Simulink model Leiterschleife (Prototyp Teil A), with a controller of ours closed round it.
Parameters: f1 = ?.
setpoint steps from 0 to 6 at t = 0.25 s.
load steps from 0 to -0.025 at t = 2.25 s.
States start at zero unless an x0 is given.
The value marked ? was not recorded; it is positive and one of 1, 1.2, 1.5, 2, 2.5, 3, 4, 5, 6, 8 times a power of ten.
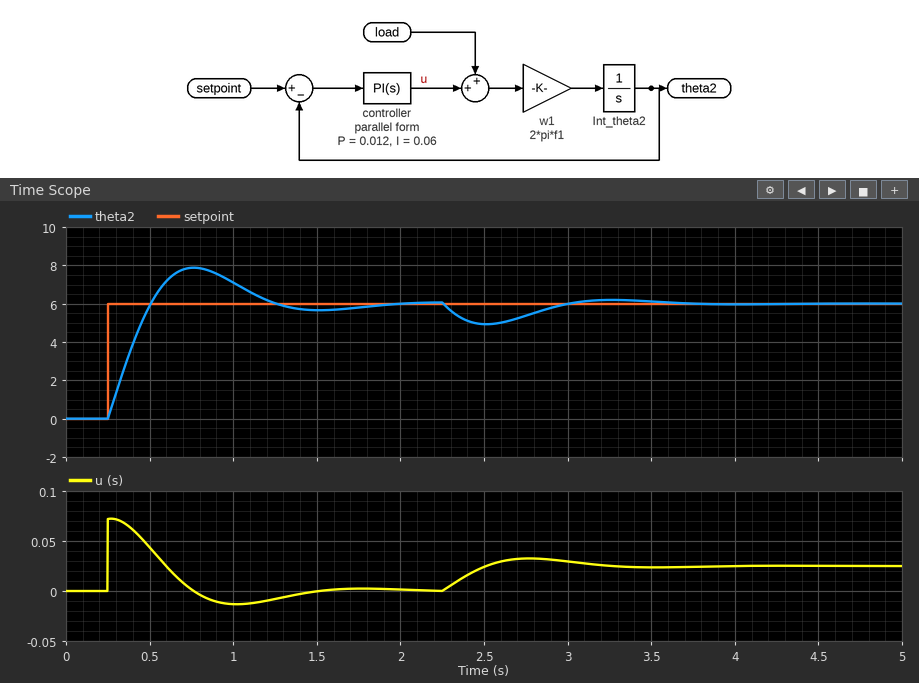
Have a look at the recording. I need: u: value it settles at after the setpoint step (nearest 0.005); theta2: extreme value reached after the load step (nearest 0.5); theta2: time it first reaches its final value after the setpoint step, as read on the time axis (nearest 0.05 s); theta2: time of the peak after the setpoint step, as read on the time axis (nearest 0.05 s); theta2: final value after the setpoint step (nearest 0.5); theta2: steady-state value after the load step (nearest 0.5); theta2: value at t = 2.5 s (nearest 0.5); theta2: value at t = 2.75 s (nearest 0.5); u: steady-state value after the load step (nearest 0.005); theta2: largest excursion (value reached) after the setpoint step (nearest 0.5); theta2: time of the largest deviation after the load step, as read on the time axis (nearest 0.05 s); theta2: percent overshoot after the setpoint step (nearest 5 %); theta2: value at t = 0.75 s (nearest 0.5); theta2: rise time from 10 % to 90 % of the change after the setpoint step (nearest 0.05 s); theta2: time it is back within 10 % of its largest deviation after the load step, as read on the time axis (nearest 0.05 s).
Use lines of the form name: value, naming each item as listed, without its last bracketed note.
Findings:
u: value it settles at after the setpoint step: 0.000
theta2: extreme value reached after the load step: 5.0
theta2: time it first reaches its final value after the setpoint step, as read on the time axis: 0.50 s
theta2: time of the peak after the setpoint step, as read on the time axis: 0.75 s
theta2: final value after the setpoint step: 6.0
theta2: steady-state value after the load step: 6.0
theta2: value at t = 2.5 s: 5.0
theta2: value at t = 2.75 s: 5.5
u: steady-state value after the load step: 0.025
theta2: largest excursion (value reached) after the setpoint step: 8.0
theta2: time of the largest deviation after the load step, as read on the time axis: 2.50 s
theta2: percent overshoot after the setpoint step: 30 %
theta2: value at t = 0.75 s: 8.0
theta2: rise time from 10 % to 90 % of the change after the setpoint step: 0.20 s
theta2: time it is back within 10 % of its largest deviation after the load step, as read on the time axis: 3.50 s
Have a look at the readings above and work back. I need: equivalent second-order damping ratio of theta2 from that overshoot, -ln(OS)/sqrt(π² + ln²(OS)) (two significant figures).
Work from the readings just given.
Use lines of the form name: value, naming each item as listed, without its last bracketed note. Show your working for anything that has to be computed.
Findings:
equivalent second-order damping ratio of theta2 from that overshoot, -ln(OS)/sqrt(π² + ln²(OS)): ln(0.3) = -1.204; 1.204 / sqrt(9.870 + 1.450) = 0.36
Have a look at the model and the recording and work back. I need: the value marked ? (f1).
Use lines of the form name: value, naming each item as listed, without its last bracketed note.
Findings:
the value marked ?: 60
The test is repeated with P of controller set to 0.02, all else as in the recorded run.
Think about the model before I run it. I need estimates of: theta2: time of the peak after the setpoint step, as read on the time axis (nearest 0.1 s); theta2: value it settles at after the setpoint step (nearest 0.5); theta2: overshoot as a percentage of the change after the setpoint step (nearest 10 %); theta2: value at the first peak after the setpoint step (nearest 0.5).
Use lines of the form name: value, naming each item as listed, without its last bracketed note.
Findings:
theta2: time of the peak after the setpoint step, as read on the time axis: 0.7 s
theta2: value it settles at after the setpoint step: 6.0
theta2: overshoot as a percentage of the change after the setpoint step: 20 %
theta2: value at the first peak after the setpoint step: 7.0
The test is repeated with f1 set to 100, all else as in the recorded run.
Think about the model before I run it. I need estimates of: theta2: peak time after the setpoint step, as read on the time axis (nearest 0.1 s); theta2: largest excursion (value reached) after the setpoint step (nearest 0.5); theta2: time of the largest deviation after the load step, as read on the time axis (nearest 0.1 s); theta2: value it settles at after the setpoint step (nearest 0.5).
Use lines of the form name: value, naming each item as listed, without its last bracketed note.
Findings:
theta2: peak time after the setpoint step, as read on the time axis: 0.6 s
theta2: largest excursion (value reached) after the setpoint step: 7.5
theta2: time of the largest deviation after the load step, as read on the time axis: 2.4 s
theta2: value it settles at after the setpoint step: 6.0
